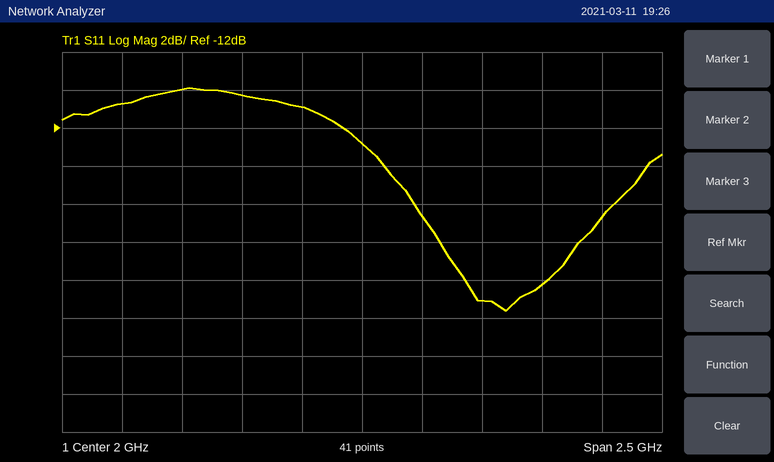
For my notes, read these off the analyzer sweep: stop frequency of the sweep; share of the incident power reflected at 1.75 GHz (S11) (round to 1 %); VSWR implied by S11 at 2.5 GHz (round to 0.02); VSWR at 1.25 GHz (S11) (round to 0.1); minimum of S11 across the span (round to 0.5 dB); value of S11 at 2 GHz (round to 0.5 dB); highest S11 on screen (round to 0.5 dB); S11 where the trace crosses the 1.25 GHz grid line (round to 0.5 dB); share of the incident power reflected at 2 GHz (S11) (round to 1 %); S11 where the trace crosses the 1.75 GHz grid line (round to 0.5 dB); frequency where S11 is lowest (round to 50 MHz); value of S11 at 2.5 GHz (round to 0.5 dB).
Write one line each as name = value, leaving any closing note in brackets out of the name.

stop frequency of the sweep = 3.25 GHz
share of the incident power reflected at 1.75 GHz (S11) = 8 %
VSWR implied by S11 at 2.5 GHz = 1.20
VSWR at 1.25 GHz (S11) = 1.9
minimum of S11 across the span = -21.5 dB
value of S11 at 2 GHz = -13.0 dB
highest S11 on screen = -10.0 dB
S11 where the trace crosses the 1.25 GHz grid line = -10.0 dB
share of the incident power reflected at 2 GHz (S11) = 5 %
S11 where the trace crosses the 1.75 GHz grid line = -11.0 dB
frequency where S11 is lowest = 2.60 GHz
value of S11 at 2.5 GHz = -21.0 dB
